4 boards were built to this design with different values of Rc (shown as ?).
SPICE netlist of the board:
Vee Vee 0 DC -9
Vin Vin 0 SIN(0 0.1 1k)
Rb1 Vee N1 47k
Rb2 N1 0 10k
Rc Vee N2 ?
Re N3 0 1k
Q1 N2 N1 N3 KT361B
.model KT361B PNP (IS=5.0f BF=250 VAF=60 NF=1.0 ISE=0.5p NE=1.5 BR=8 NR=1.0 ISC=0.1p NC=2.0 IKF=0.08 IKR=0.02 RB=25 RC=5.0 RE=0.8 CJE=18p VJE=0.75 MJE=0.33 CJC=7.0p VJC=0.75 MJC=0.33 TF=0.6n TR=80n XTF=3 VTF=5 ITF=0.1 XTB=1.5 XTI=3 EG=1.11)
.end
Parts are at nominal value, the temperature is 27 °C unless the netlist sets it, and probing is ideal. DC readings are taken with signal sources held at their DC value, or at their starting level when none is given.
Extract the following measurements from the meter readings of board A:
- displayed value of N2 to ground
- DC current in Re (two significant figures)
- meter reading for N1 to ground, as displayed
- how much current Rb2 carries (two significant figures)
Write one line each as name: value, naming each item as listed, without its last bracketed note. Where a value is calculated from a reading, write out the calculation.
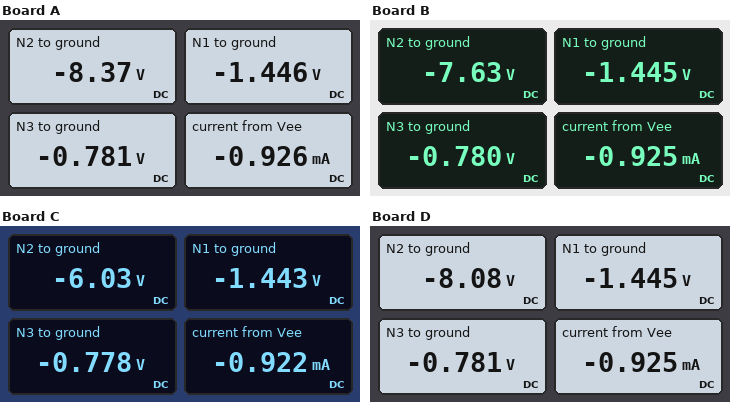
displayed value of N2 to ground: -8.37 V
DC current in Re: (0 V - (-781 mV)) / 1 kΩ = 780 µA
meter reading for N1 to ground, as displayed: -1.446 V
how much current Rb2 carries: (0 V - (-1.446 V)) / 10 kΩ = 140 µA
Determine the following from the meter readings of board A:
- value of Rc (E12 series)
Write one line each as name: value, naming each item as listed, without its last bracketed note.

value of Rc: 820 Ω
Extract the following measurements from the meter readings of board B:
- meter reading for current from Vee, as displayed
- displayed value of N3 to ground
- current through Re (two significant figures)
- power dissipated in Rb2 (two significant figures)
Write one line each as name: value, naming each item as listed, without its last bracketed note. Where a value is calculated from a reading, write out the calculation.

meter reading for current from Vee, as displayed: -0.925 mA
displayed value of N3 to ground: -0.780 V
current through Re: (0 V - (-780 mV)) / 1 kΩ = 780 µA
power dissipated in Rb2: (0 V - (-1.445 V))^2 / 10 kΩ = 210 µW
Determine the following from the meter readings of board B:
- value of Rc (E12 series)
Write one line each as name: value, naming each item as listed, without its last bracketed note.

value of Rc: 1.8 kΩ
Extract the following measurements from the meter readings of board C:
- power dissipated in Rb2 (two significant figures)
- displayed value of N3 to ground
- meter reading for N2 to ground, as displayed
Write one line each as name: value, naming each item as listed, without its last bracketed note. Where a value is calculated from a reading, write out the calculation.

power dissipated in Rb2: (0 V - (-1.443 V))^2 / 10 kΩ = 210 µW
displayed value of N3 to ground: -0.778 V
meter reading for N2 to ground, as displayed: -6.03 V
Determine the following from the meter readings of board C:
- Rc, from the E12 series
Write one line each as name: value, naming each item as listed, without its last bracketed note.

Rc, from the E12 series: 3.9 kΩ
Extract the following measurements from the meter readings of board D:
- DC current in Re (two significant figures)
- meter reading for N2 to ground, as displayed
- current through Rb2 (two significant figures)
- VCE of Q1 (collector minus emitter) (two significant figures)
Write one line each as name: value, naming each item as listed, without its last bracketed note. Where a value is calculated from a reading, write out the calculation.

DC current in Re: (0 V - (-781 mV)) / 1 kΩ = 780 µA
meter reading for N2 to ground, as displayed: -8.08 V
current through Rb2: (0 V - (-1.445 V)) / 10 kΩ = 140 µA
VCE of Q1 (collector minus emitter): -8.08 V - (-781 mV) = -7.3 V
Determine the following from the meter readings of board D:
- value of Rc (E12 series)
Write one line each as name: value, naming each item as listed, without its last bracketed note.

value of Rc: 1.2 kΩ
